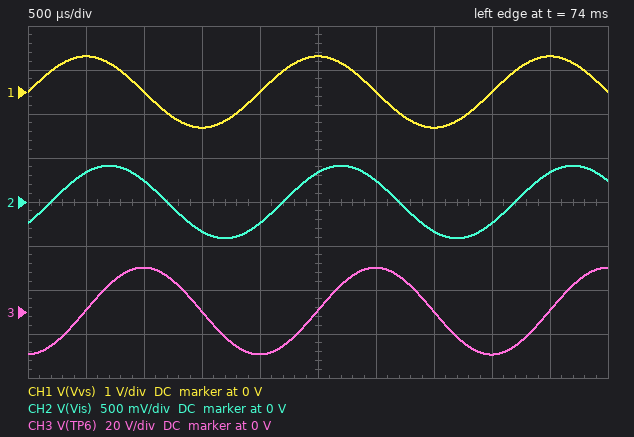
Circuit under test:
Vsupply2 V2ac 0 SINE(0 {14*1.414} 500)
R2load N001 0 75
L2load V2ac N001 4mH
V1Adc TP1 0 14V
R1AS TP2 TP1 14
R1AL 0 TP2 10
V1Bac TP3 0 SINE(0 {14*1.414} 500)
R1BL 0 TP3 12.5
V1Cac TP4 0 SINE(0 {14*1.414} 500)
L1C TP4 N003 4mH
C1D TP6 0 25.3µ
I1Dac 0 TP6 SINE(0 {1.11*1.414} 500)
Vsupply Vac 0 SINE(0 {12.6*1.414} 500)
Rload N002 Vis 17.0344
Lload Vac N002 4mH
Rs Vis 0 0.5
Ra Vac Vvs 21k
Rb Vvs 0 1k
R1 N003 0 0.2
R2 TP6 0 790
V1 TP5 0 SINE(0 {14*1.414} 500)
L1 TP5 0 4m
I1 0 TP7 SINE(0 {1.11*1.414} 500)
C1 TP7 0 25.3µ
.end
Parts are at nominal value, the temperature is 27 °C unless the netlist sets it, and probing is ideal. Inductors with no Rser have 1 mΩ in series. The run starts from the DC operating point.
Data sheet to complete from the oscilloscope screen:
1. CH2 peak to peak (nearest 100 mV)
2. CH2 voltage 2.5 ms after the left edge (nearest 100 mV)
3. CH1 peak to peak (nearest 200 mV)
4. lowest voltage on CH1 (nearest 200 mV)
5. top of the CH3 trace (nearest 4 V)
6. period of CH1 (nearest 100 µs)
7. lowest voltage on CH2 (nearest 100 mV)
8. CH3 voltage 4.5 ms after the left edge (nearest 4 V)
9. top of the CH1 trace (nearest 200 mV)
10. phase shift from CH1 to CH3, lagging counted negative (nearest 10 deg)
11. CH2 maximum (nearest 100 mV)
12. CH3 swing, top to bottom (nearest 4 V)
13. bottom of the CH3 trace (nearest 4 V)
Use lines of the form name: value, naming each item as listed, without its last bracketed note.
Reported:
CH2 peak to peak: 800 mV
CH2 voltage 2.5 ms after the left edge: 300 mV
CH1 peak to peak: 1.6 V
lowest voltage on CH1: -800 mV
top of the CH3 trace: 20 V
period of CH1: 2.0 ms
lowest voltage on CH2: -400 mV
CH3 voltage 4.5 ms after the left edge: 0 V
top of the CH1 trace: 800 mV
phase shift from CH1 to CH3, lagging counted negative: -90 deg
CH2 maximum: 400 mV
CH3 swing, top to bottom: 40 V
bottom of the CH3 trace: -20 V
